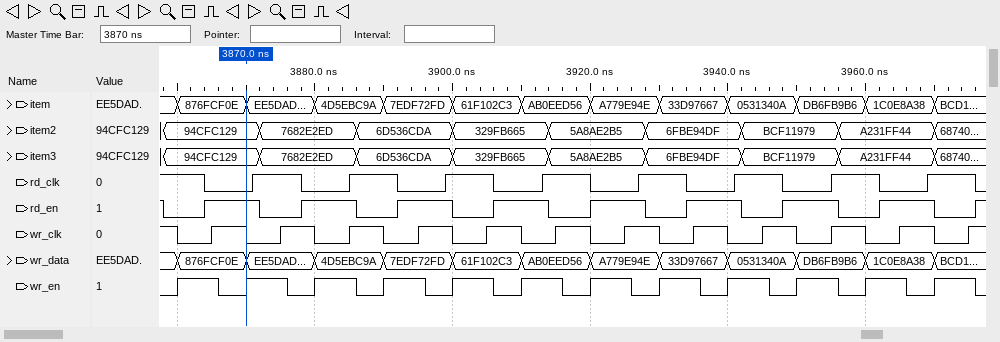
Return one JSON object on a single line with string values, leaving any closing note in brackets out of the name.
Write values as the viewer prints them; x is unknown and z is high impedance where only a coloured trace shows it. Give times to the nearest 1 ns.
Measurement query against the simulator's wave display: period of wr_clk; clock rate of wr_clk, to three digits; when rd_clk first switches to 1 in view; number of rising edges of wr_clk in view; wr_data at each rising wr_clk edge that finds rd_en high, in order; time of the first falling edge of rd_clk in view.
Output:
{"period of wr_clk": "10 ns", "clock rate of wr_clk, to three digits": "100 MHz", "when rd_clk first switches to 1 in view": "3871 ns", "number of rising edges of wr_clk in view": "12", "wr_data at each rising wr_clk edge that finds rd_en high, in order": "876FCF0E, 4D5EBC9A, 7EDF72FD, A779E94E, 33D97667, DB6FB9B6, 1C0E8A38", "time of the first falling edge of rd_clk in view": "3864 ns"}
